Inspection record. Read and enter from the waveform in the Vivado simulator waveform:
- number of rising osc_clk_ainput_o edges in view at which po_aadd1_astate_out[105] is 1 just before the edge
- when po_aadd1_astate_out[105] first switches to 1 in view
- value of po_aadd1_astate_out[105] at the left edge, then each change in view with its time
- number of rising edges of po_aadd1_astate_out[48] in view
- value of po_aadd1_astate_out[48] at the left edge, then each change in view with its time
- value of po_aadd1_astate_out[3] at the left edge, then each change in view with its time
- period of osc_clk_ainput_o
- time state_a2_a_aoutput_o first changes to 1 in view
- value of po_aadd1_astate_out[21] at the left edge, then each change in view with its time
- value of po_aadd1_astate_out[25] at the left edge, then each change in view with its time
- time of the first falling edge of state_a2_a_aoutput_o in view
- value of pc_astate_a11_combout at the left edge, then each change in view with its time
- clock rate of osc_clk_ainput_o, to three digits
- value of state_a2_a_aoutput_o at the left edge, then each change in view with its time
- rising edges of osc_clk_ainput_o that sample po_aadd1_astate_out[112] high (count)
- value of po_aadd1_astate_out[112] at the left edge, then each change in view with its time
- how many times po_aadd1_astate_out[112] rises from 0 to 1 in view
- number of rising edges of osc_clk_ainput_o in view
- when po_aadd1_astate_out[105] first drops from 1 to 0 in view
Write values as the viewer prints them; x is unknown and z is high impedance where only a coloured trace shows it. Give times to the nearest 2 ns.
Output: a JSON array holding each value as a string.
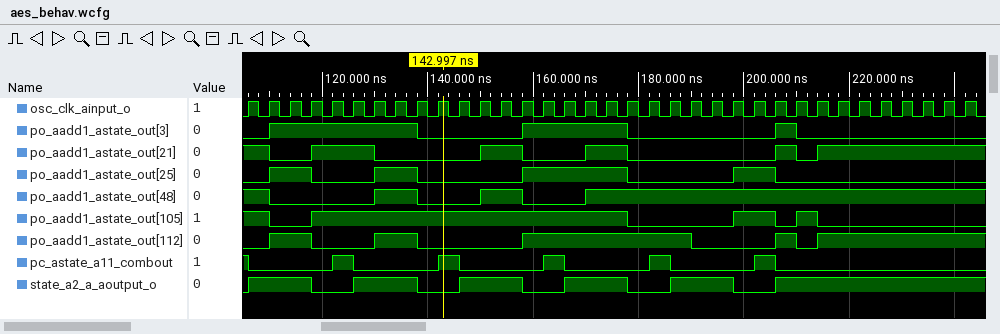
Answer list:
["20", "118 ns", "1, 0 at 110 ns, 1 at 118 ns, 0 at 178 ns, 1 at 198 ns, 0 at 206 ns, 1 at 210 ns, 0 at 214 ns", "3", "1, 0 at 110 ns, 1 at 130 ns, 0 at 138 ns, 1 at 150 ns, 0 at 158 ns, 1 at 170 ns", "0, 1 at 110 ns, 0 at 138 ns, 1 at 158 ns, 0 at 178 ns, 1 at 206 ns, 0 at 210 ns", "4 ns", "106 ns", "1, 0 at 110 ns, 1 at 118 ns, 0 at 130 ns, 1 at 150 ns, 0 at 158 ns, 1 at 170 ns, 0 at 178 ns, 1 at 206 ns, 0 at 210 ns, 1 at 214 ns", "0, 1 at 110 ns, 0 at 118 ns, 1 at 130 ns, 0 at 138 ns, 1 at 158 ns, 0 at 178 ns, 1 at 198 ns, 0 at 206 ns", "118 ns", "1, 0 at 106 ns, 1 at 122 ns, 0 at 126 ns, 1 at 142 ns, 0 at 146 ns, 1 at 162 ns, 0 at 166 ns, 1 at 182 ns, 0 at 186 ns, 1 at 202 ns, 0 at 206 ns", "250 MHz", "0, 1 at 106 ns, 0 at 118 ns, 1 at 126 ns, 0 at 138 ns, 1 at 146 ns, 0 at 158 ns, 1 at 166 ns, 0 at 178 ns, 1 at 186 ns, 0 at 198 ns, 1 at 206 ns", "20", "0, 1 at 110 ns, 0 at 118 ns, 1 at 130 ns, 0 at 138 ns, 1 at 158 ns, 0 at 190 ns, 1 at 206 ns, 0 at 210 ns, 1 at 214 ns", "5", "35", "110 ns"]
